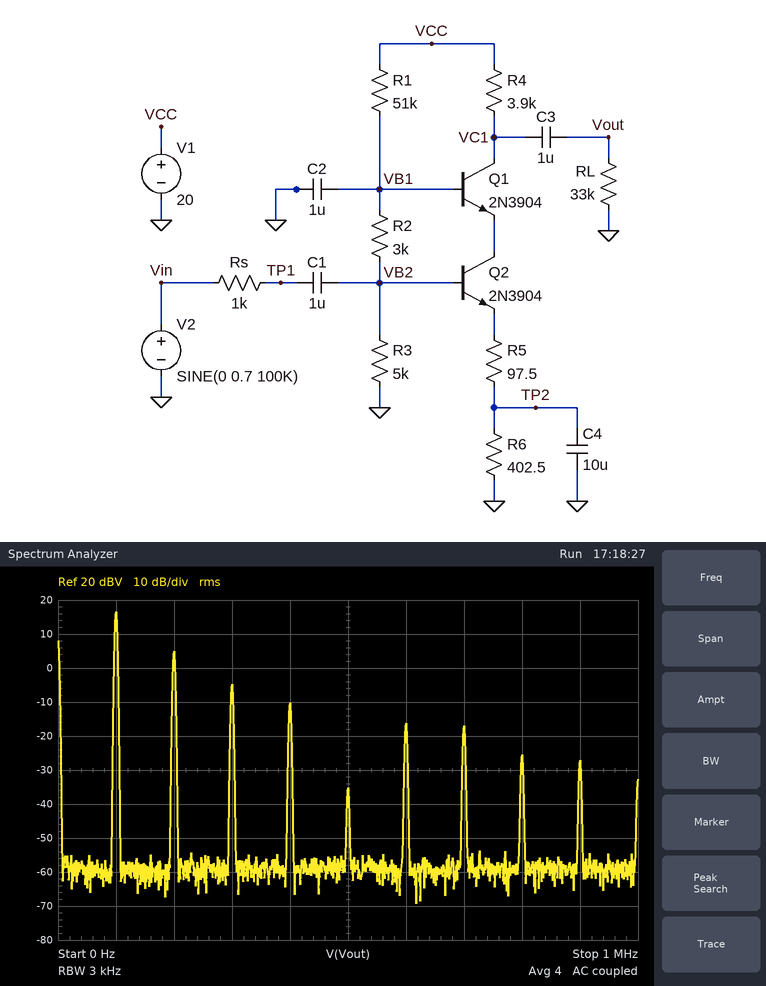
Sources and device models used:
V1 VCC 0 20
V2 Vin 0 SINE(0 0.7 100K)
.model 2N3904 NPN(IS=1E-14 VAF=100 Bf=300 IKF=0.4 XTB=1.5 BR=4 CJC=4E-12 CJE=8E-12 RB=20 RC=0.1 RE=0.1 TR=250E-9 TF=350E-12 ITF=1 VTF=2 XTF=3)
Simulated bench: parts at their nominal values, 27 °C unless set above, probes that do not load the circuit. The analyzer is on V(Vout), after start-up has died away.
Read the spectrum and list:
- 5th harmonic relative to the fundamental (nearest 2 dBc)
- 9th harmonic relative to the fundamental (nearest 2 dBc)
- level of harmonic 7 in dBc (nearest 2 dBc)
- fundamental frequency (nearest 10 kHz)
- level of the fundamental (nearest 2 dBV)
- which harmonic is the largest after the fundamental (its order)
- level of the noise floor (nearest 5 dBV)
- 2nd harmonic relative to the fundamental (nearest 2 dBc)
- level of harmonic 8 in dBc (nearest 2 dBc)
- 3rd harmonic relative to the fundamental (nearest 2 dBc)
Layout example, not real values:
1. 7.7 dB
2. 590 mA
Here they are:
1. -52 dBc
2. -44 dBc
3. -34 dBc
4. 100 kHz
5. 16 dBV
6. 2
7. -60 dBV
8. -12 dBc
9. -42 dBc
10. -22 dBc
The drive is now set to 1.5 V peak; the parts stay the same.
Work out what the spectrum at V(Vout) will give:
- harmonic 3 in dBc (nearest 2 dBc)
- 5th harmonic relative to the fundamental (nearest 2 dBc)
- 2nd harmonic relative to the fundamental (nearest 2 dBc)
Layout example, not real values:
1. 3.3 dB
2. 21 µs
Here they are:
1. -20 dBc
2. -22 dBc
3. -8 dBc
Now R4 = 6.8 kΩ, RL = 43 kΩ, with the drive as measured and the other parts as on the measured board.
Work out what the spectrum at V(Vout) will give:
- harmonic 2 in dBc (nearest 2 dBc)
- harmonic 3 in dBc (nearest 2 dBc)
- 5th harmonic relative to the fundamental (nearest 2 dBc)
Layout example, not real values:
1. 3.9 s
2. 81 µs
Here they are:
1. -10 dBc
2. -16 dBc
3. -28 dBc
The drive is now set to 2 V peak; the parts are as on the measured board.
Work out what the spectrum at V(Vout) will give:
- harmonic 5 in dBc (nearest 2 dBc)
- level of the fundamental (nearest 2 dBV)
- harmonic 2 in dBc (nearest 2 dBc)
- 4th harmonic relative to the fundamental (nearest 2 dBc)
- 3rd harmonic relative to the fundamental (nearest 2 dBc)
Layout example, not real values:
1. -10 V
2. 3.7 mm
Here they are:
1. -28 dBc
2. 18 dBV
3. -10 dBc
4. -12 dBc
5. -16 dBc
